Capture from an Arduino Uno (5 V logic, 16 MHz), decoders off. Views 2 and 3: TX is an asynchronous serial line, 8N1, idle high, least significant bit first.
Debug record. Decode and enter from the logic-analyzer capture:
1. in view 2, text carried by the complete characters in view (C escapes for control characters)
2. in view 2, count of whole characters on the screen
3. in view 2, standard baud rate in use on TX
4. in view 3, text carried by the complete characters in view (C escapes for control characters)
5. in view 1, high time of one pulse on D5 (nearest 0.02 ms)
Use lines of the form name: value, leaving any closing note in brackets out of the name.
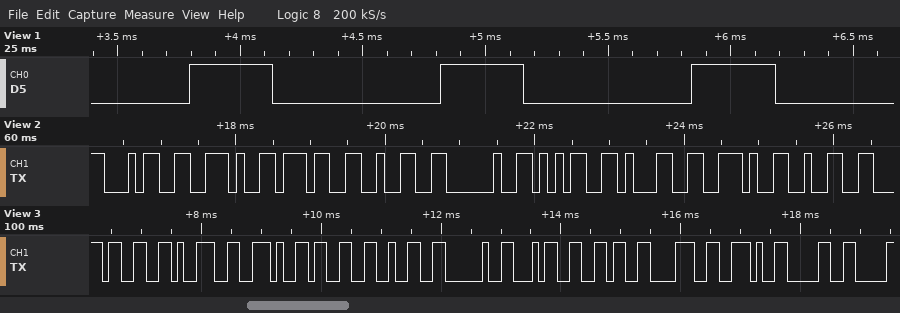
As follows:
in view 2, text carried by the complete characters in view: "4.72 51.2"
in view 2, count of whole characters on the screen: 9
in view 2, standard baud rate in use on TX: 9600 baud
in view 3, text carried by the complete characters in view: "39.32 468.0"
in view 1, high time of one pulse on D5: 0.34 ms
